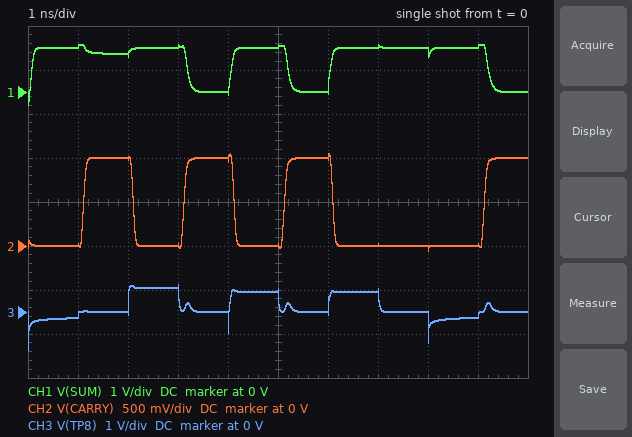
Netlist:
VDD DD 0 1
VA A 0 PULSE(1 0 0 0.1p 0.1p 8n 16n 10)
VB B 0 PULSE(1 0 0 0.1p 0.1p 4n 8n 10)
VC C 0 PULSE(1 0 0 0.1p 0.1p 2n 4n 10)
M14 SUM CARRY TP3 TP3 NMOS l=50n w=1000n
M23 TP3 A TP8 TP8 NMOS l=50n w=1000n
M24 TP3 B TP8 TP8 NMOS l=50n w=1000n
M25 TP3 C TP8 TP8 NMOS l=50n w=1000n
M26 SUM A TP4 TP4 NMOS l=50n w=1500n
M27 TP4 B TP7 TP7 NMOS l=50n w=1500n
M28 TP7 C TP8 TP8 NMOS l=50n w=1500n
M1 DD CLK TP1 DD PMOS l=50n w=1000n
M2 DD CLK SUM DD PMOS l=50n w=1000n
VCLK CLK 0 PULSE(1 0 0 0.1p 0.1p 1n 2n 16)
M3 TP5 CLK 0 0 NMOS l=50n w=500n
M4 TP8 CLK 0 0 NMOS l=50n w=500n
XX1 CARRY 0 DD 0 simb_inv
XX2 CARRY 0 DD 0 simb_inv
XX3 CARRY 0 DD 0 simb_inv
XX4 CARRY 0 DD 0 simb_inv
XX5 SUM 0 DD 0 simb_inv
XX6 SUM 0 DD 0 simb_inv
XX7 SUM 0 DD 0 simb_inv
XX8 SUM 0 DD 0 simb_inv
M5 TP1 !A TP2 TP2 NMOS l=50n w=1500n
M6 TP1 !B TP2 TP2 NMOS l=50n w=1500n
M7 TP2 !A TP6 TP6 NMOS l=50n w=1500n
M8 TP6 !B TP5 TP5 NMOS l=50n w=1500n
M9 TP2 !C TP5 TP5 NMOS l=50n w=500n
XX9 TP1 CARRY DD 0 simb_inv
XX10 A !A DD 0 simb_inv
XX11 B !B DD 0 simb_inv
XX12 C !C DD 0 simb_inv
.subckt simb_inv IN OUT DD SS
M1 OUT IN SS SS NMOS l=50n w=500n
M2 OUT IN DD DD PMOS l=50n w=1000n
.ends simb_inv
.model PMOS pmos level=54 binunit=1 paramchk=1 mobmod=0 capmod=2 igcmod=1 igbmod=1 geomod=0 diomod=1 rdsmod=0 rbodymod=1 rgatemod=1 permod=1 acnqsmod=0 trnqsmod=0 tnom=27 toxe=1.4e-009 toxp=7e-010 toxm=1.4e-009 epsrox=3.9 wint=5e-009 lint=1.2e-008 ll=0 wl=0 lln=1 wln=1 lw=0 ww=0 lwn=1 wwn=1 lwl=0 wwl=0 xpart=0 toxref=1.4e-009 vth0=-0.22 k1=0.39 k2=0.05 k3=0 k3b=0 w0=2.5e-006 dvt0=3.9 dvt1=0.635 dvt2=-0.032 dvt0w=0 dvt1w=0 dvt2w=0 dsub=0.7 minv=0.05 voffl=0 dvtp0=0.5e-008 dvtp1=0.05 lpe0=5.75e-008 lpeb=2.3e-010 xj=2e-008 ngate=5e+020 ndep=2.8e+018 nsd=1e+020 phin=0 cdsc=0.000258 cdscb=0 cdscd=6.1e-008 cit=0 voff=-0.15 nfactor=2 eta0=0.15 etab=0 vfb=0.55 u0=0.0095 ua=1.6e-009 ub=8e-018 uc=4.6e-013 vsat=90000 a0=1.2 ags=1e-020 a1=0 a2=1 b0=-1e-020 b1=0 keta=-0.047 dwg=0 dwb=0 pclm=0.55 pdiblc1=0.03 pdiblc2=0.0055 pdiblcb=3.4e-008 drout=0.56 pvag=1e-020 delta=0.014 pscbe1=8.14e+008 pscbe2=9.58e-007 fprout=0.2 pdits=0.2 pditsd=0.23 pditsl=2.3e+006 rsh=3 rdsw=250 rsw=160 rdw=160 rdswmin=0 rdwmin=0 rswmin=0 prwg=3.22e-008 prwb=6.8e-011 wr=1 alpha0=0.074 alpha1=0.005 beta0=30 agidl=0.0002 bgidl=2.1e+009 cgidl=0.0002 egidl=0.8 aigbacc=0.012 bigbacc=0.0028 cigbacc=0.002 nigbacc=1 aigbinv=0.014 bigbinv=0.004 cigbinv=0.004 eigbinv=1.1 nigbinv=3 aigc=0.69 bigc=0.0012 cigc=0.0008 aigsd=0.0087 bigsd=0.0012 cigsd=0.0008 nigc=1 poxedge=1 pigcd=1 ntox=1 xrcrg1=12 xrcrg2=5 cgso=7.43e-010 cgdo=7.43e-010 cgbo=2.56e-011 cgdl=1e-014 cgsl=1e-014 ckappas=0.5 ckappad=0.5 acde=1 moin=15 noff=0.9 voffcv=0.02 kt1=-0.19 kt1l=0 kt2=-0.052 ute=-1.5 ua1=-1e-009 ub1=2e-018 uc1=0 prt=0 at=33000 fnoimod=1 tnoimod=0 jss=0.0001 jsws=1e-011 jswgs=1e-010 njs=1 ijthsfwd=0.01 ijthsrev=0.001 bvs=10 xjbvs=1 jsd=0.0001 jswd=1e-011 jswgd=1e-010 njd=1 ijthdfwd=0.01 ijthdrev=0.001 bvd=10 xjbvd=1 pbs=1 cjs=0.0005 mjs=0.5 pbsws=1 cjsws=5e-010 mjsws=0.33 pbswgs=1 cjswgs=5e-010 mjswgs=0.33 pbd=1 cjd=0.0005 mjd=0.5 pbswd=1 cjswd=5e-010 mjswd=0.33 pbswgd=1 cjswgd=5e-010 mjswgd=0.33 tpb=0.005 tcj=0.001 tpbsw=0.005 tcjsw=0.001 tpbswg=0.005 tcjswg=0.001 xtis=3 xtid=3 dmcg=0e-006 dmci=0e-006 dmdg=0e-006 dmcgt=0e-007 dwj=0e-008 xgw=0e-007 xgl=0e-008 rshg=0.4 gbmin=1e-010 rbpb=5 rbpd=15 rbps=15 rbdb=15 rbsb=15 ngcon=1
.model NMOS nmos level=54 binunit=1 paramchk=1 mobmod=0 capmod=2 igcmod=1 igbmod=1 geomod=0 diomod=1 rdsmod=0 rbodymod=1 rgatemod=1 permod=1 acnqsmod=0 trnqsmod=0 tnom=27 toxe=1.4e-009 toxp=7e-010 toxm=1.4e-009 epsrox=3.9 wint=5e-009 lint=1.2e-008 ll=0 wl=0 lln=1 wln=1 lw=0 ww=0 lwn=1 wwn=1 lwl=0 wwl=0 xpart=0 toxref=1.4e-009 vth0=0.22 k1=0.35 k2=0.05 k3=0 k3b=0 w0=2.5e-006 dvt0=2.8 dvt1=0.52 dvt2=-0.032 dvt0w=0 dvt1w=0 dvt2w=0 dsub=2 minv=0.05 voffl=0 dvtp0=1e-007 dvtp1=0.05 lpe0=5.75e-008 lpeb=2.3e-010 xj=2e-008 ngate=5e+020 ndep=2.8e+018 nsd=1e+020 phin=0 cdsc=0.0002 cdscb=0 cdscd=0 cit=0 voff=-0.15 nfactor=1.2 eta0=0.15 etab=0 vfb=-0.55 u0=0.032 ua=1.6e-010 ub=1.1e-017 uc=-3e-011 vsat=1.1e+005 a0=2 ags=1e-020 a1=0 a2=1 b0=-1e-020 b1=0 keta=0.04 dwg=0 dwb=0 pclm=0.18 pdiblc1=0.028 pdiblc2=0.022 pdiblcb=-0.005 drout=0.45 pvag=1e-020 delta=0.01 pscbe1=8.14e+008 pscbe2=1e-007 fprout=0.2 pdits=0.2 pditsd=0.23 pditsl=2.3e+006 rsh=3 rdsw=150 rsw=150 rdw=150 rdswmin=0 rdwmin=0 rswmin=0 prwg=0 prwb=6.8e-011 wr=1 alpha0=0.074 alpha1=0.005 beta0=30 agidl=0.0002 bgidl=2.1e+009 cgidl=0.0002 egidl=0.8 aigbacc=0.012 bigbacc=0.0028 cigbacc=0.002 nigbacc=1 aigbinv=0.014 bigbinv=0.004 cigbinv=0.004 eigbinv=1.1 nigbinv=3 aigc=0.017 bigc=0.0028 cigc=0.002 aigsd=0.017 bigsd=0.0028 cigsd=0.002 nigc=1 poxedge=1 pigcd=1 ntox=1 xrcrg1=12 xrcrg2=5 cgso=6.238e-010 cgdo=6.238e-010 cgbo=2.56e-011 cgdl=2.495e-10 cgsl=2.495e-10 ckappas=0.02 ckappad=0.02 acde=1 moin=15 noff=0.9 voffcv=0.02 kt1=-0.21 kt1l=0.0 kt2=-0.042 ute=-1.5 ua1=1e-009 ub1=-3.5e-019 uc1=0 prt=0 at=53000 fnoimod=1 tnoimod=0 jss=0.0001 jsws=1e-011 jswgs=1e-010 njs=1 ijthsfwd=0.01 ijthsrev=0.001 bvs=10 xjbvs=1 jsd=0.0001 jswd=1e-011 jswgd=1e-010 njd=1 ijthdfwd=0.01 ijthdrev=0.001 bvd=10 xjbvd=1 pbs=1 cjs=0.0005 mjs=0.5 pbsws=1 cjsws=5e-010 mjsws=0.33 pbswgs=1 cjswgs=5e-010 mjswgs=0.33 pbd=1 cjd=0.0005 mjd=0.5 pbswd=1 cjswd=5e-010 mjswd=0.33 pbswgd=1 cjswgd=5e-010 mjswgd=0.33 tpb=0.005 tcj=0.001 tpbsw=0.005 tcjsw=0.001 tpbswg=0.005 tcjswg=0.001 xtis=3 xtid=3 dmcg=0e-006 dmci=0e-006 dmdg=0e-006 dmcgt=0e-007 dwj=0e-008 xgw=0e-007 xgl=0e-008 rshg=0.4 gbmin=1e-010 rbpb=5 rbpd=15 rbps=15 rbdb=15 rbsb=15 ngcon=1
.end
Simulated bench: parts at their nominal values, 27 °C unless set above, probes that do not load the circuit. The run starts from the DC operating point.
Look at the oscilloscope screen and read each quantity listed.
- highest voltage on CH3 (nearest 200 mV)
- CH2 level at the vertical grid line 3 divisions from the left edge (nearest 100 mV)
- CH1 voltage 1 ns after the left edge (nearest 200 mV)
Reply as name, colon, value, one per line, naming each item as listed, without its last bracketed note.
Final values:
highest voltage on CH3: 600 mV
CH2 level at the vertical grid line 3 divisions from the left edge: 0 V
CH1 voltage 1 ns after the left edge: 1.0 V
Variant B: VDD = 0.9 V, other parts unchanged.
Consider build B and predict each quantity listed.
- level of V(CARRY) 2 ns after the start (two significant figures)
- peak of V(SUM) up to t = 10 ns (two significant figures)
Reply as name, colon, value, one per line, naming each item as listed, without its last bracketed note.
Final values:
level of V(CARRY) 2 ns after the start: 900 mV
peak of V(SUM) up to t = 10 ns: 970 mV
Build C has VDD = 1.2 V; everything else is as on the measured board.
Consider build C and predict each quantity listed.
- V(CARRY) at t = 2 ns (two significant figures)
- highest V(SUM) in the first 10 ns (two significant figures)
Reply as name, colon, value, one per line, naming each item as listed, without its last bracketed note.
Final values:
V(CARRY) at t = 2 ns: 1.2 V
highest V(SUM) in the first 10 ns: 1.3 V
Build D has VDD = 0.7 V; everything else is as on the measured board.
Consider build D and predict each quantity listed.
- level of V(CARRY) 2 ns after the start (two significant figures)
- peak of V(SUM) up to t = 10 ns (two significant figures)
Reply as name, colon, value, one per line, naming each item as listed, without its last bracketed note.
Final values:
level of V(CARRY) 2 ns after the start: 700 mV
peak of V(SUM) up to t = 10 ns: 760 mV
